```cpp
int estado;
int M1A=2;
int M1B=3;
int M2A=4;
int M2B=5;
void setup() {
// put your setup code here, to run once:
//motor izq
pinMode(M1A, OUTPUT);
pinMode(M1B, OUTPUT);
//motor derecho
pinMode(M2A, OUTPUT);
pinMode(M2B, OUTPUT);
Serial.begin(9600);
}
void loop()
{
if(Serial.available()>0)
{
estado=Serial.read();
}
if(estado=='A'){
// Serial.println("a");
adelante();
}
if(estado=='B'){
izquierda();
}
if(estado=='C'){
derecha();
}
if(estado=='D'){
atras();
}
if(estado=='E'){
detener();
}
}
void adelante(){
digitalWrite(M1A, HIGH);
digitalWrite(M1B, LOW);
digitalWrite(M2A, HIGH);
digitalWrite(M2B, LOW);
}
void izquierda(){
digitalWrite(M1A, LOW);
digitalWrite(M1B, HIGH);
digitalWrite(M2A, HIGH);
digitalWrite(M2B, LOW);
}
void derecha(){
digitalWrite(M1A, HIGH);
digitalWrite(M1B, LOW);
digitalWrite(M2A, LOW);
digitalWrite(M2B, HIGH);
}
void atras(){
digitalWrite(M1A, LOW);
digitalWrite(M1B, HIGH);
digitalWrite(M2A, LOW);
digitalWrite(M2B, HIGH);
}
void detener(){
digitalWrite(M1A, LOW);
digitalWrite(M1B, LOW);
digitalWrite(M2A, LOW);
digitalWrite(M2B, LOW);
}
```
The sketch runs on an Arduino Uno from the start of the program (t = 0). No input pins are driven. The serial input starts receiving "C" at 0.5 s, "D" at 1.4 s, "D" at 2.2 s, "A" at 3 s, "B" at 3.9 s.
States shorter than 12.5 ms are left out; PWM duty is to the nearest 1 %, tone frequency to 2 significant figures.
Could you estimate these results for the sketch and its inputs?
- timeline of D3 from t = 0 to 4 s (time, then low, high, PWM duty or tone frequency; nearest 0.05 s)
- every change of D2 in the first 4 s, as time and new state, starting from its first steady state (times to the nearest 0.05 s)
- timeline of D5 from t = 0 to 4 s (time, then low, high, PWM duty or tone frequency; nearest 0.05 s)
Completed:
0 s low; 1.4 s high; 3 s low; 3.9 s high
0 s low; 0.5 s high; 1.4 s low; 3 s high; 3.9 s low
0 s low; 0.5 s high; 3 s low
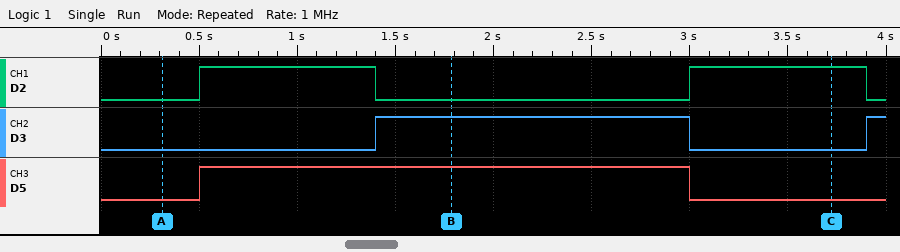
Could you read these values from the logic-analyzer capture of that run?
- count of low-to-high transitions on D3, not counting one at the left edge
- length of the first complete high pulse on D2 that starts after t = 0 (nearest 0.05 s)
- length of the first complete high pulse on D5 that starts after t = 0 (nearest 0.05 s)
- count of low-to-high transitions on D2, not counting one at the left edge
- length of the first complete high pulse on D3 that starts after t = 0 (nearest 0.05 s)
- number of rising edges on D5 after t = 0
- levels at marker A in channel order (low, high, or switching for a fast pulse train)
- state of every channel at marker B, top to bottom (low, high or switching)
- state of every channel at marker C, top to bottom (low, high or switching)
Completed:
2
0.90 s
2.50 s
2
1.60 s
1
D2 low, D3 low, D5 low
D2 low, D3 high, D5 high
D2 high, D3 low, D5 low
